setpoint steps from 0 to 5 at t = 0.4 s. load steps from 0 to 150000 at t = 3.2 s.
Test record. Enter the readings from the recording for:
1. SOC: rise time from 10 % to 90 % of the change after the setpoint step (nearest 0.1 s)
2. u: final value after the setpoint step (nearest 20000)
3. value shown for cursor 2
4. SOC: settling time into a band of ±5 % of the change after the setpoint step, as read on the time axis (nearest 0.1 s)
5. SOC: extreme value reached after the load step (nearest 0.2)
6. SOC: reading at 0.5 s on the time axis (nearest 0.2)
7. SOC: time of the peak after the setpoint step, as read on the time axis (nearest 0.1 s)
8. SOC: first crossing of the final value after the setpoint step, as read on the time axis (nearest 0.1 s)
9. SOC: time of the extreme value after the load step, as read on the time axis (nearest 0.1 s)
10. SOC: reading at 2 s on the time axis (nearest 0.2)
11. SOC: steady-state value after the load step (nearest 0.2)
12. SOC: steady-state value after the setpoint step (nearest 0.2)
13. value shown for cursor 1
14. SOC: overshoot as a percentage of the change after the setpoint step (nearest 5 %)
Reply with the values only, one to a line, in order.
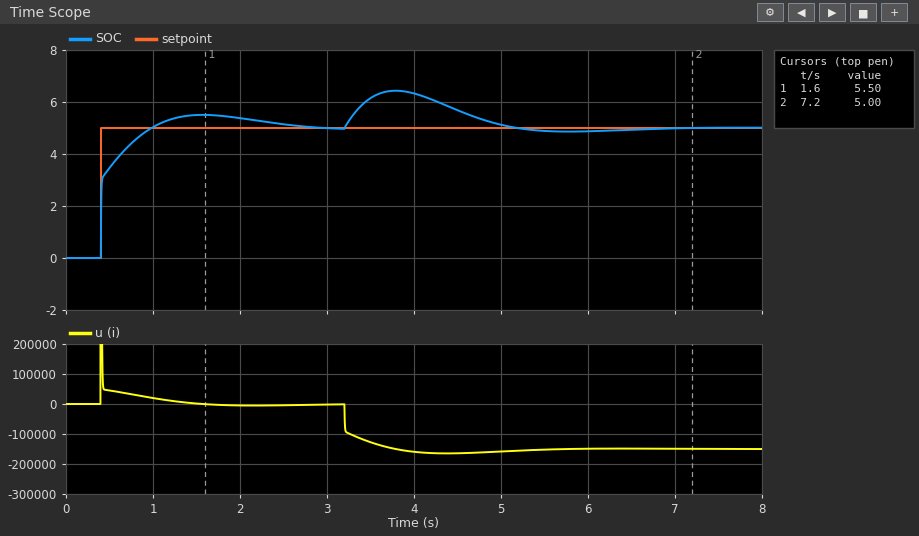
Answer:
0.4 s
0
5.00
2.3 s
6.4
3.4
1.6 s
1.0 s
3.8 s
5.4
5.0
5.0
5.50
10 %
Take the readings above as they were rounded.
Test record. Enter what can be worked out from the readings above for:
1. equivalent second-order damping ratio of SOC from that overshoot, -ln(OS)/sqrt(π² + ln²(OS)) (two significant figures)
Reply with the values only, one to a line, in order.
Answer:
0.59
